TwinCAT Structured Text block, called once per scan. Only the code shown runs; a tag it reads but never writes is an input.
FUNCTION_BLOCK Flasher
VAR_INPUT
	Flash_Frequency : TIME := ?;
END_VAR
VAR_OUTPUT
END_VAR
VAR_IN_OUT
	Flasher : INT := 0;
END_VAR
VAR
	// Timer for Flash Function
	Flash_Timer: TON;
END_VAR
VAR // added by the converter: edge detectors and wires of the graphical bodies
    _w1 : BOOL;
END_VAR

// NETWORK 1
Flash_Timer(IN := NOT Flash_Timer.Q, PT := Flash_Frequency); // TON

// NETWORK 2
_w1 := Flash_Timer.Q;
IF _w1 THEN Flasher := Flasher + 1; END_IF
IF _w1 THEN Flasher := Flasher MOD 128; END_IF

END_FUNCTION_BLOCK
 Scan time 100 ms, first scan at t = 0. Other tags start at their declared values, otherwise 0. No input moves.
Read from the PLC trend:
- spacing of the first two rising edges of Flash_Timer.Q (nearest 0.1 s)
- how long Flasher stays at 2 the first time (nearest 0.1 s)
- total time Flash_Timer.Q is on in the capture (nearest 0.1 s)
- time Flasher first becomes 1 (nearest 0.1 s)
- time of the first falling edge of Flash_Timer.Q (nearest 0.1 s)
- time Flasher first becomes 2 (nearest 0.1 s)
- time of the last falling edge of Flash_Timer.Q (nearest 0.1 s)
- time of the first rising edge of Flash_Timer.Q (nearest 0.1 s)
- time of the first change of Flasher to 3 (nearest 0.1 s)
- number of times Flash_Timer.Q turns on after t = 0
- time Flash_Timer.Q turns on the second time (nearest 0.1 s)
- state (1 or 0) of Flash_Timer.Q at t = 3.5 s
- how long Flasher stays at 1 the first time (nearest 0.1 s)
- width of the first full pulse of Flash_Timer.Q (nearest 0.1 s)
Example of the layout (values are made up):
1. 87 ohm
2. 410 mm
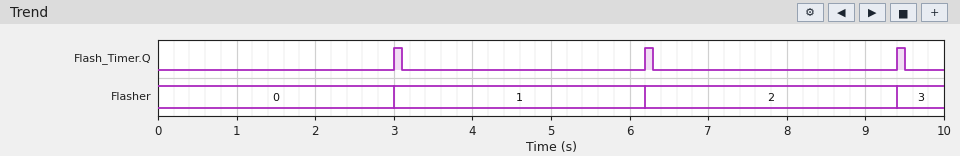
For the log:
1. 3.2 s
2. 3.2 s
3. 0.3 s
4. 3.0 s
5. 3.1 s
6. 6.2 s
7. 9.5 s
8. 3.0 s
9. 9.4 s
10. 3
11. 6.2 s
12. 0
13. 3.2 s
14. 0.1 s
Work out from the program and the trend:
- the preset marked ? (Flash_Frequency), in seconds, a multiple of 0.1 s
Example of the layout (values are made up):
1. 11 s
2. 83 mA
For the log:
1. 3.0 s
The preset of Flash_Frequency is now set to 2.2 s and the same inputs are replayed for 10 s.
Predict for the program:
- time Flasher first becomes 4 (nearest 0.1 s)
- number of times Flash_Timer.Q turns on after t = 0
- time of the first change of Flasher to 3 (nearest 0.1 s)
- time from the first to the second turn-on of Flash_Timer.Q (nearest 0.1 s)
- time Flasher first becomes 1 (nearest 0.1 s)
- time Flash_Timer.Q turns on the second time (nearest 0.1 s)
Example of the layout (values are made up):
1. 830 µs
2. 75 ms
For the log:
1. 9.4 s
2. 4
3. 7.0 s
4. 2.4 s
5. 2.2 s
6. 4.6 s
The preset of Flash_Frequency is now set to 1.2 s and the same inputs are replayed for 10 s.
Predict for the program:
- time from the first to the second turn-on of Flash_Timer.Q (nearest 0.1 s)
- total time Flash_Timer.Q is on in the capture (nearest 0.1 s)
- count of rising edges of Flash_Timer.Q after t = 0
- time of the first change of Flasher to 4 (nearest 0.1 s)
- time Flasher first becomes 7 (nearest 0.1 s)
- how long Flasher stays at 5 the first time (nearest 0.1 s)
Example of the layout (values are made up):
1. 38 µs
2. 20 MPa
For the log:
1. 1.4 s
2. 0.7 s
3. 7
4. 5.4 s
5. 9.6 s
6. 1.4 s
